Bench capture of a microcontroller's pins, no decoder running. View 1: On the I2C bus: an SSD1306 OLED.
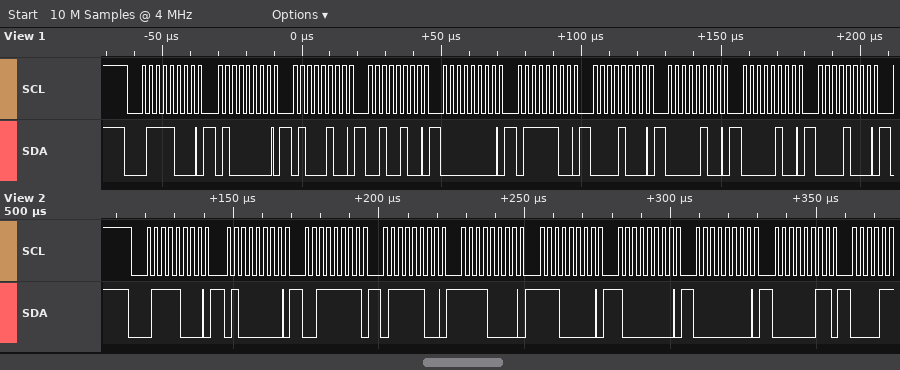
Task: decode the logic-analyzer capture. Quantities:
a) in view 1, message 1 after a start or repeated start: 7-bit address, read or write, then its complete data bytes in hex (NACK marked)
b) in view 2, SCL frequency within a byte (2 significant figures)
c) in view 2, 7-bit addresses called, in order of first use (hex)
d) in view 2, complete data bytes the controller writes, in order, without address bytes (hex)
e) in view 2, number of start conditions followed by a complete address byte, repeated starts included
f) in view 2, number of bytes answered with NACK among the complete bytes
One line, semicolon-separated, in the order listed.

0x3C write: 40 44 24 00 7C 08 04 04 08; 400 kHz; 0x3C; 40 3F 7C F0 E0 80 00 03; 1; 0
